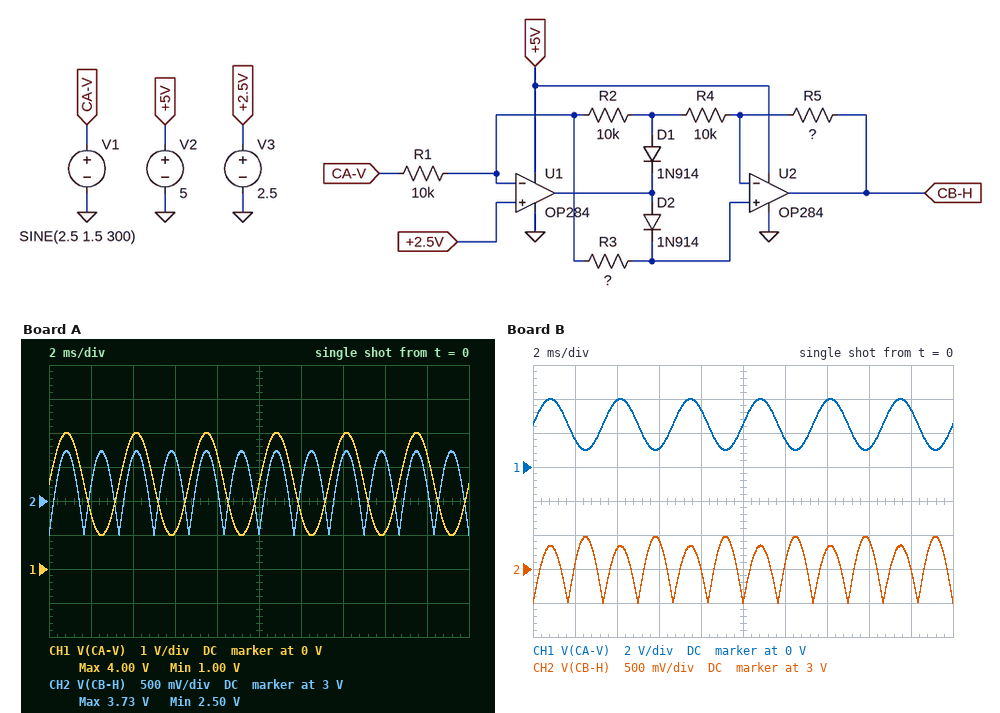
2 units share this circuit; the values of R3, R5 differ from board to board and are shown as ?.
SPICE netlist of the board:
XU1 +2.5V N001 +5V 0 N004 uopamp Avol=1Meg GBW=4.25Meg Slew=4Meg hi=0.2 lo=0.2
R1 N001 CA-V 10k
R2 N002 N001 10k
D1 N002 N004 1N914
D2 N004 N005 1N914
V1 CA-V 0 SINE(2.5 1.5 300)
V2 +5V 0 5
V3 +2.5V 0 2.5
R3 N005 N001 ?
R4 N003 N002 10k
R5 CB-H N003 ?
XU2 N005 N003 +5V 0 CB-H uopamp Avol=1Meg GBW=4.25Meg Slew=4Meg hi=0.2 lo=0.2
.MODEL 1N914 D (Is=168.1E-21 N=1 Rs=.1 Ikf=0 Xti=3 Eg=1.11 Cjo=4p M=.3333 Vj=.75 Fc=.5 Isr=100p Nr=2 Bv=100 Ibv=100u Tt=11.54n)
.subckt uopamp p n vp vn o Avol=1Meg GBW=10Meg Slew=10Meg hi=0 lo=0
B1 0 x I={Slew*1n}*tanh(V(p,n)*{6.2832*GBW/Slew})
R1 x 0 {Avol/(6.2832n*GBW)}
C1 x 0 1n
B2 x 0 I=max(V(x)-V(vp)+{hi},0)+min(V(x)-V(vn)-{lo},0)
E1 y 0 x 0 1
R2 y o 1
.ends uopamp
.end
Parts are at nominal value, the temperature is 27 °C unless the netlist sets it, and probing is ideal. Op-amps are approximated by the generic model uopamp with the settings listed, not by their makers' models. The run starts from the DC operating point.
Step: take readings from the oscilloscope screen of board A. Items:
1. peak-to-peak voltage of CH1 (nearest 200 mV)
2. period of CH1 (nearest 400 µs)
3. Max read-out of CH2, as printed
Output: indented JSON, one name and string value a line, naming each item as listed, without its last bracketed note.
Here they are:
{
  "peak-to-peak voltage of CH1": "3.0 V",
  "period of CH1": "3.2 ms",
  "Max read-out of CH2, as printed": "3.73 V"
}
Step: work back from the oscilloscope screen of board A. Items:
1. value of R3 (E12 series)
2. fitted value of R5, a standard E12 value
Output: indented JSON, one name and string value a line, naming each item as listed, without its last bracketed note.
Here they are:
{
  "value of R3": "8.2 kΩ",
  "fitted value of R5, a standard E12 value": "8.2 kΩ"
}
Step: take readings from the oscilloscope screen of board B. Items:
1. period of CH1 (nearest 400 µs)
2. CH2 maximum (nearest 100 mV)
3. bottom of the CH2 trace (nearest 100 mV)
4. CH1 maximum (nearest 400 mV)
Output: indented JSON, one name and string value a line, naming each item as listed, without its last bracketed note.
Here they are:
{
  "period of CH1": "3.2 ms",
  "CH2 maximum": "3.5 V",
  "bottom of the CH2 trace": "2.5 V",
  "CH1 maximum": "4.0 V"
}
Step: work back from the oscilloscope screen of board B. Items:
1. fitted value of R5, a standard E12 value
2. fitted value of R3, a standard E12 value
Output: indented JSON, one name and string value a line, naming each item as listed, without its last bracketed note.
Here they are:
{
  "fitted value of R5, a standard E12 value": "5.6 kΩ",
  "fitted value of R3, a standard E12 value": "6.8 kΩ"
}
